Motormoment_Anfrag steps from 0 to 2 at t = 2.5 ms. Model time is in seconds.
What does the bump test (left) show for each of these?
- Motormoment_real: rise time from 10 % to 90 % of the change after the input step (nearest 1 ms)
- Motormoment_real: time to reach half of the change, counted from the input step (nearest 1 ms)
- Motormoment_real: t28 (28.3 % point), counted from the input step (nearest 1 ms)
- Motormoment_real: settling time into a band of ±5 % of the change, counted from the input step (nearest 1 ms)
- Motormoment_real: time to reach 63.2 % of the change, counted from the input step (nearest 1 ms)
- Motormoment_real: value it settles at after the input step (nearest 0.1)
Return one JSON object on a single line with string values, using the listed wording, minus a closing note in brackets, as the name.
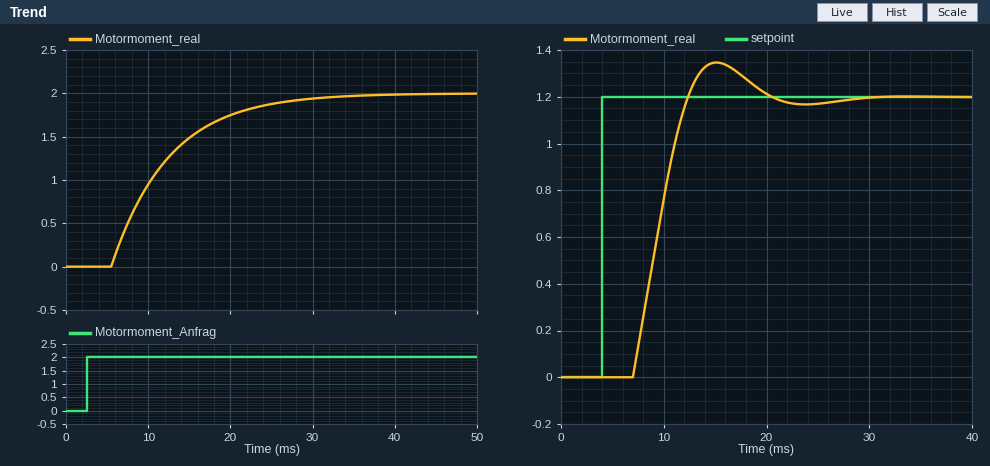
{"Motormoment_real: rise time from 10 % to 90 % of the change after the input step": "15 ms", "Motormoment_real: time to reach half of the change, counted from the input step": "8 ms", "Motormoment_real: t28 (28.3 % point), counted from the input step": "5 ms", "Motormoment_real: settling time into a band of ±5 % of the change, counted from the input step": "24 ms", "Motormoment_real: time to reach 63.2 % of the change, counted from the input step": "10 ms", "Motormoment_real: value it settles at after the input step": "2.0"}
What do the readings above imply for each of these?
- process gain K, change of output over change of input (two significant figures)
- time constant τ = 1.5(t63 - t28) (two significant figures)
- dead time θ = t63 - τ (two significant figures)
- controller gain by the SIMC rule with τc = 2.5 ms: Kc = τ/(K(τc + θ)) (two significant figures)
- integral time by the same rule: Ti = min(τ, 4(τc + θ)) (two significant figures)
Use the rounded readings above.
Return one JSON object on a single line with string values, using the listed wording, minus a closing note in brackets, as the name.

{"process gain K, change of output over change of input": "1.0", "time constant τ = 1.5(t63 - t28)": "7.5 ms", "dead time θ = t63 - τ": "2.5 ms", "controller gain by the SIMC rule with τc = 2.5 ms: Kc = τ/(K(τc + θ))": "1.5", "integral time by the same rule: Ti = min(τ, 4(τc + θ))": "7.5 ms"}
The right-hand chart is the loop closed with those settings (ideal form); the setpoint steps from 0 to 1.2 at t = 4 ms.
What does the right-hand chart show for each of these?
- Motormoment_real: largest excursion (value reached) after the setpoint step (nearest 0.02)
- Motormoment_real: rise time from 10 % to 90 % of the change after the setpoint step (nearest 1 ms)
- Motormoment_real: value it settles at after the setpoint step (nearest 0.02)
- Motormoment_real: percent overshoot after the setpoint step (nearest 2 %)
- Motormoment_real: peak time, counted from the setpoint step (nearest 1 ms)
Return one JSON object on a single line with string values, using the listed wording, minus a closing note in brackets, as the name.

{"Motormoment_real: largest excursion (value reached) after the setpoint step": "1.34", "Motormoment_real: rise time from 10 % to 90 % of the change after the setpoint step": "4 ms", "Motormoment_real: value it settles at after the setpoint step": "1.20", "Motormoment_real: percent overshoot after the setpoint step": "12 %", "Motormoment_real: peak time, counted from the setpoint step": "11 ms"}
